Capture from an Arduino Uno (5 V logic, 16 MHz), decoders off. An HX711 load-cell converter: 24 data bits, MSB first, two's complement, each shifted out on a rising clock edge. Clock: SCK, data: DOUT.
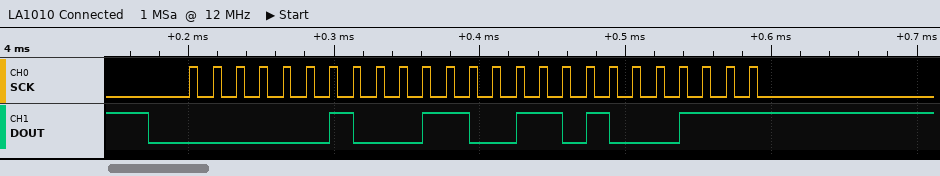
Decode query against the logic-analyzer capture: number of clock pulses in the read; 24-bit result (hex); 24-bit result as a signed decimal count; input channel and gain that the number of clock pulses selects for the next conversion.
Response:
25
0x023347
144199
channel A, gain 128
